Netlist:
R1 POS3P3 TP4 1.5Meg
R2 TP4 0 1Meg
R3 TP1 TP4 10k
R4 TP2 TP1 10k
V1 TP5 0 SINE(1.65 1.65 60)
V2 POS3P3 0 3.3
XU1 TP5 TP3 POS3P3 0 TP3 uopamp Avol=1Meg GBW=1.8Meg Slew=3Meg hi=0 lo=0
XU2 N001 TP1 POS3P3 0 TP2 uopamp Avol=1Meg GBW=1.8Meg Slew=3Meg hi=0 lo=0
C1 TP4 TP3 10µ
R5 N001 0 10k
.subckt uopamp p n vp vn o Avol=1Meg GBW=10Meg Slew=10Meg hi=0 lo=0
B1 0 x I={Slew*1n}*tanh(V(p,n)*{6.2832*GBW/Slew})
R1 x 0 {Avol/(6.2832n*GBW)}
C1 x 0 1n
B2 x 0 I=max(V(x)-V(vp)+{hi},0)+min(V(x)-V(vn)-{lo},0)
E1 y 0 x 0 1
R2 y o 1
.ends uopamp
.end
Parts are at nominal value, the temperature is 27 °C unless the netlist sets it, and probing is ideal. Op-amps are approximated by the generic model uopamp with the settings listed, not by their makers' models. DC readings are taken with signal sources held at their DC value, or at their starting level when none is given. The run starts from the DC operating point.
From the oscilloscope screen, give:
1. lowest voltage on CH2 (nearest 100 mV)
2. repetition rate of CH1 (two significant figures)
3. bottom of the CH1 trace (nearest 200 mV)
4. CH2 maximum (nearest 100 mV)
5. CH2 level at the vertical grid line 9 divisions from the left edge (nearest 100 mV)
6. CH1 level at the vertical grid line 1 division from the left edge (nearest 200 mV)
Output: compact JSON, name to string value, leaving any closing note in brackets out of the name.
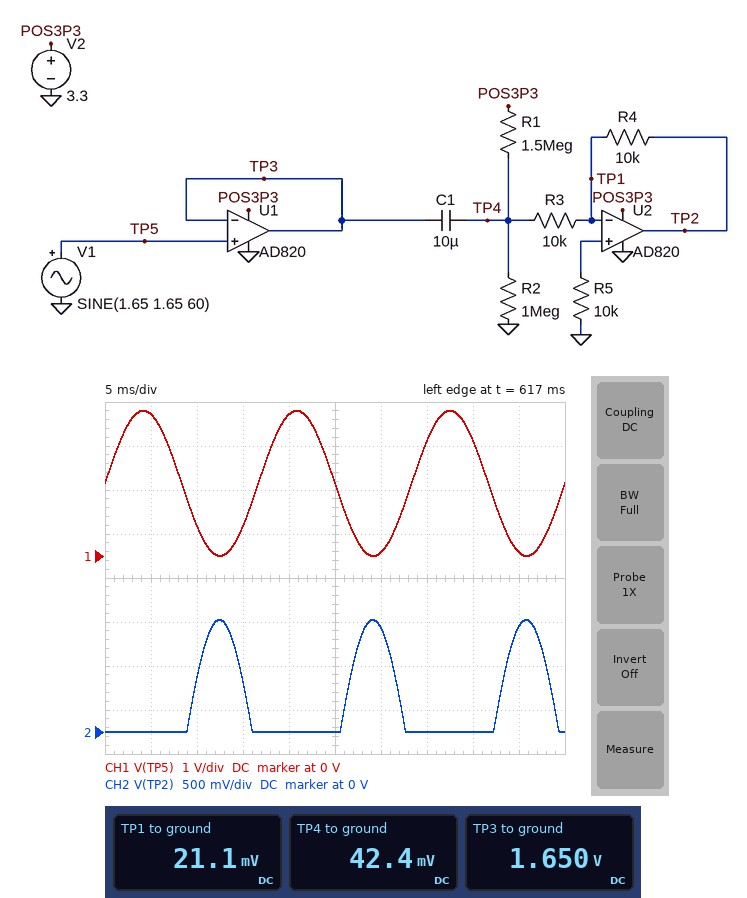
{"lowest voltage on CH2": "0 V", "repetition rate of CH1": "60 Hz", "bottom of the CH1 trace": "0 V", "CH2 maximum": "1.3 V", "CH2 level at the vertical grid line 9 divisions from the left edge": "1.2 V", "CH1 level at the vertical grid line 1 division from the left edge": "3.2 V"}
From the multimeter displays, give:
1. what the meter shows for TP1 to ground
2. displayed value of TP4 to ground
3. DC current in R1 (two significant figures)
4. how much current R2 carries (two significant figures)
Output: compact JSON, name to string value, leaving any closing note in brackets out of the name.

{"what the meter shows for TP1 to ground": "21.1 mV", "displayed value of TP4 to ground": "42.4 mV", "DC current in R1": "2.2 µA", "how much current R2 carries": "42 nA"}
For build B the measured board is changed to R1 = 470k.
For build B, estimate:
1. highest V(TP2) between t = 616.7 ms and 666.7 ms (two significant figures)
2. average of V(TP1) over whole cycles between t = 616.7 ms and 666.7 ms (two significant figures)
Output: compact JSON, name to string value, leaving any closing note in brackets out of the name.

{"highest V(TP2) between t = 616.7 ms and 666.7 ms": "1.2 V", "average of V(TP1) over whole cycles between t = 616.7 ms and 666.7 ms": "380 mV"}
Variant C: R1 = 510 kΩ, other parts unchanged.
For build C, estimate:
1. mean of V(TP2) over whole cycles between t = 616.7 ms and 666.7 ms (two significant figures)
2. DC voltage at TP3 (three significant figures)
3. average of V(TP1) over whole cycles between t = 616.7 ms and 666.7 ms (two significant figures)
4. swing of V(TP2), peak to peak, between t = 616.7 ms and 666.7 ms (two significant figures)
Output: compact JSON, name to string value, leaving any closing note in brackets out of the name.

{"mean of V(TP2) over whole cycles between t = 616.7 ms and 666.7 ms": "330 mV", "DC voltage at TP3": "1.65 V", "average of V(TP1) over whole cycles between t = 616.7 ms and 666.7 ms": "380 mV", "swing of V(TP2), peak to peak, between t = 616.7 ms and 666.7 ms": "1.2 V"}
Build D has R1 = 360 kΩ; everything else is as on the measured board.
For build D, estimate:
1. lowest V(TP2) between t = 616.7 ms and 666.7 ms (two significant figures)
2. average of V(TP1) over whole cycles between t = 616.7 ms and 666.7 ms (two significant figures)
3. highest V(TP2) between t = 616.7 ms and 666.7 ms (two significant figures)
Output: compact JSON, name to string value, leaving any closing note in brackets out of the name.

{"lowest V(TP2) between t = 616.7 ms and 666.7 ms": "-2.9 mV", "average of V(TP1) over whole cycles between t = 616.7 ms and 666.7 ms": "390 mV", "highest V(TP2) between t = 616.7 ms and 666.7 ms": "1.2 V"}
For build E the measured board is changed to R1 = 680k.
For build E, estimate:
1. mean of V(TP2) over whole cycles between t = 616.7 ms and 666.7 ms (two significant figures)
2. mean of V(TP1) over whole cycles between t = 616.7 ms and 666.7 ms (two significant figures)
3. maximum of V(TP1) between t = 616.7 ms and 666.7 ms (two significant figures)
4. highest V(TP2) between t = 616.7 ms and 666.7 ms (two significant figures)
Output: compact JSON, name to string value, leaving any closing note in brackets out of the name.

{"mean of V(TP2) over whole cycles between t = 616.7 ms and 666.7 ms": "340 mV", "mean of V(TP1) over whole cycles between t = 616.7 ms and 666.7 ms": "370 mV", "maximum of V(TP1) between t = 616.7 ms and 666.7 ms": "1.0 V", "highest V(TP2) between t = 616.7 ms and 666.7 ms": "1.2 V"}
